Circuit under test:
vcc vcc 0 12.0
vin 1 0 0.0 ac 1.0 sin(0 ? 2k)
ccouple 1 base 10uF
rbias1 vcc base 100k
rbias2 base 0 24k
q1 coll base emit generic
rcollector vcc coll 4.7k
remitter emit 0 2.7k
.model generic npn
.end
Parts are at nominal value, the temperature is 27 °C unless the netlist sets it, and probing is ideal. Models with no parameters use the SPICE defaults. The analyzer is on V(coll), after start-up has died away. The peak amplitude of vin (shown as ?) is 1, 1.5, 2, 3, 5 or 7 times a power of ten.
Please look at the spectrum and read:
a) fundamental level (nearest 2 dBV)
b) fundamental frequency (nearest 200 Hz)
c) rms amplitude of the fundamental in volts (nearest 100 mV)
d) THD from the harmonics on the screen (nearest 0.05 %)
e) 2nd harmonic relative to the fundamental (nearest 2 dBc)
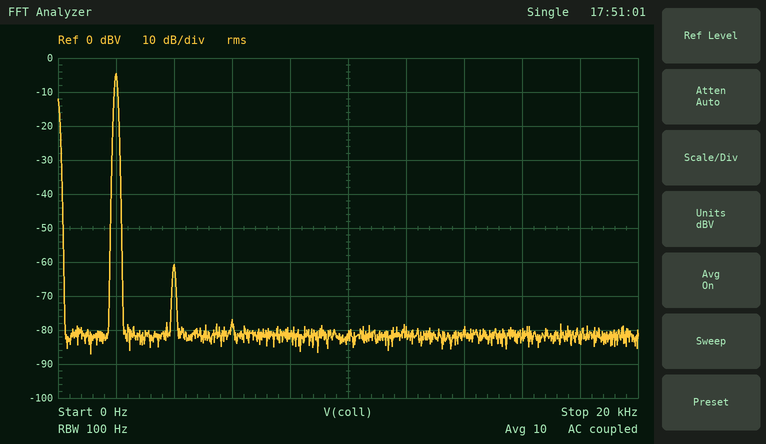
-4 dBV
2.0 kHz
600 mV
0.15 %
-56 dBc
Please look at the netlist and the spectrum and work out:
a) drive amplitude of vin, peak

500 mV
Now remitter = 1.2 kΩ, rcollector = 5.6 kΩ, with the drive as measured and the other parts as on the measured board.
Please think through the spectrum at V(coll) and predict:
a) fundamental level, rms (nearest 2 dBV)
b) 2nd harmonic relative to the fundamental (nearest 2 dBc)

4 dBV
-54 dBc
